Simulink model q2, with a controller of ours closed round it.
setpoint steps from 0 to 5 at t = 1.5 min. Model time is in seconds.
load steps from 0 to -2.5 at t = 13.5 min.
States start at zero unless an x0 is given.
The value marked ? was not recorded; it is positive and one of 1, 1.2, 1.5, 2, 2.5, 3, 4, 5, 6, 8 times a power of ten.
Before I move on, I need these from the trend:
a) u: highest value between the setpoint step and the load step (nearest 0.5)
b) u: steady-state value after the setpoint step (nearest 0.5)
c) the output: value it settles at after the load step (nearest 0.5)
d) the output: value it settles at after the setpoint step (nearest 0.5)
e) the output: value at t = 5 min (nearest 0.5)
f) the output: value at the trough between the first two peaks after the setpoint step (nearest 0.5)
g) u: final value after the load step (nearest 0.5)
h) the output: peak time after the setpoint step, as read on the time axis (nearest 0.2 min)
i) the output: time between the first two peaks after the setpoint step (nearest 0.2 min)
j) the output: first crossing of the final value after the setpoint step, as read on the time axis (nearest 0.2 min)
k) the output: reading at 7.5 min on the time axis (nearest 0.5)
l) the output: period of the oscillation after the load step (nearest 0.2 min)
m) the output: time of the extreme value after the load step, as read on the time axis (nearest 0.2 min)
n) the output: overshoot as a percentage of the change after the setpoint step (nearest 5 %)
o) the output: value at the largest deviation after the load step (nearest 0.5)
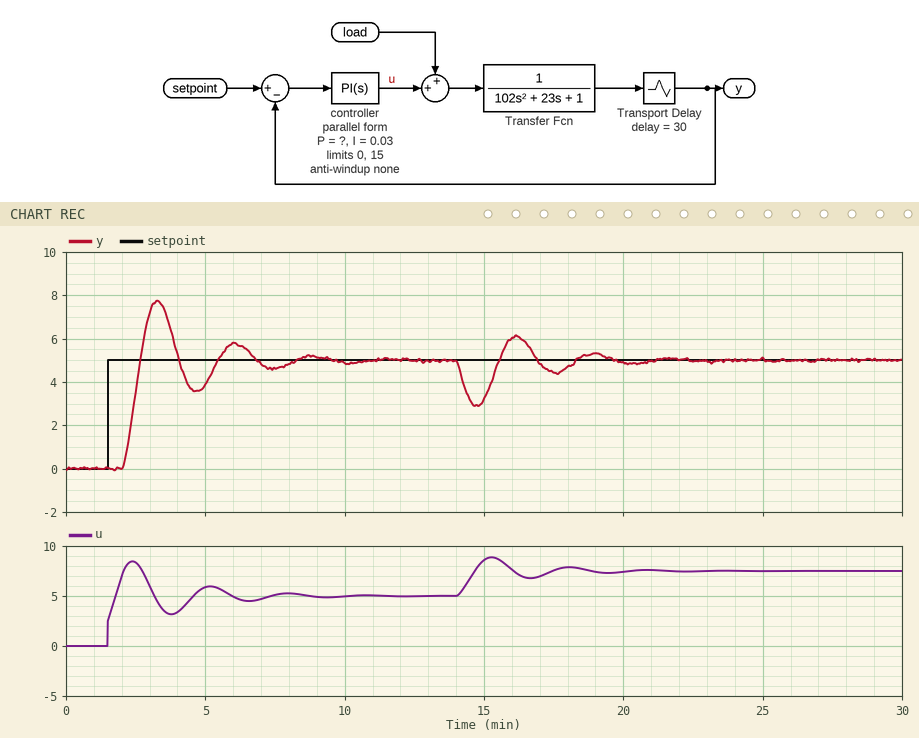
8.5
5.0
5.0
5.0
4.0
3.5
7.5
3.2 min
2.8 min
2.6 min
4.5
2.8 min
14.8 min
55 %
3.0
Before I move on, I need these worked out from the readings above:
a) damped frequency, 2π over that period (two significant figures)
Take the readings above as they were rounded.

2.2 rad/min
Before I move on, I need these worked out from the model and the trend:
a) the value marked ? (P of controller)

0.5
